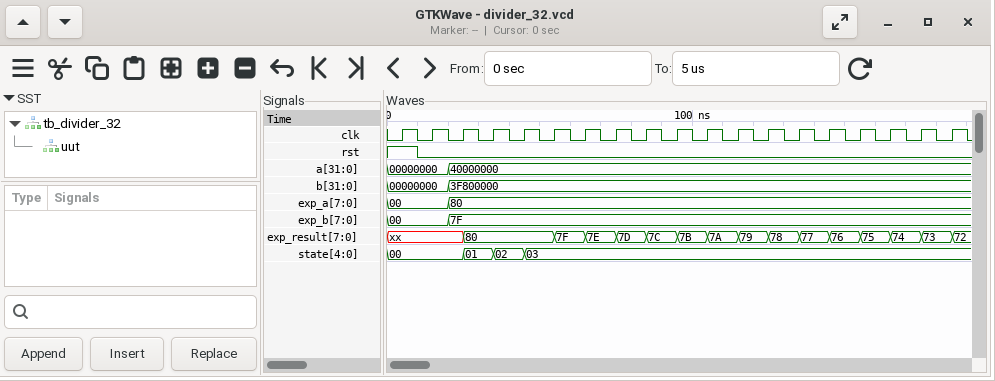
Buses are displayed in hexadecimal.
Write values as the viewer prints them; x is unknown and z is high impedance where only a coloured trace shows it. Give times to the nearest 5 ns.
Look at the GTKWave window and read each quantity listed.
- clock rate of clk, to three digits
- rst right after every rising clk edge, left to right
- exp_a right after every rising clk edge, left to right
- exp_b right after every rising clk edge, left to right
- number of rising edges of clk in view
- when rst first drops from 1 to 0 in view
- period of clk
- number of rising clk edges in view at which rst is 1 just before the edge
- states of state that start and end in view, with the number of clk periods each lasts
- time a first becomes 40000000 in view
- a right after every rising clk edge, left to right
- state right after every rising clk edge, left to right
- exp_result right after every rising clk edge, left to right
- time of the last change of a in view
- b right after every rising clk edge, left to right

100 MHz
1 0 0 0 0 0 0 0 0 0 0 0 0 0 0 0 0 0 0
00, 00, 80, 80, 80, 80, 80, 80, 80, 80, 80, 80, 80, 80, 80, 80, 80, 80, 80
00, 00, 7F, 7F, 7F, 7F, 7F, 7F, 7F, 7F, 7F, 7F, 7F, 7F, 7F, 7F, 7F, 7F, 7F
19
10 ns
10 ns
1
01: 1, 02: 1
20 ns
00000000, 00000000, 40000000, 40000000, 40000000, 40000000, 40000000, 40000000, 40000000, 40000000, 40000000, 40000000, 40000000, 40000000, 40000000, 40000000, 40000000, 40000000, 40000000
00, 00, 01, 02, 03, 03, 03, 03, 03, 03, 03, 03, 03, 03, 03, 03, 03, 03, 03
xx, xx, 80, 80, 80, 7F, 7E, 7D, 7C, 7B, 7A, 79, 78, 77, 76, 75, 74, 73, 72
20 ns
00000000, 00000000, 3F800000, 3F800000, 3F800000, 3F800000, 3F800000, 3F800000, 3F800000, 3F800000, 3F800000, 3F800000, 3F800000, 3F800000, 3F800000, 3F800000, 3F800000, 3F800000, 3F800000
